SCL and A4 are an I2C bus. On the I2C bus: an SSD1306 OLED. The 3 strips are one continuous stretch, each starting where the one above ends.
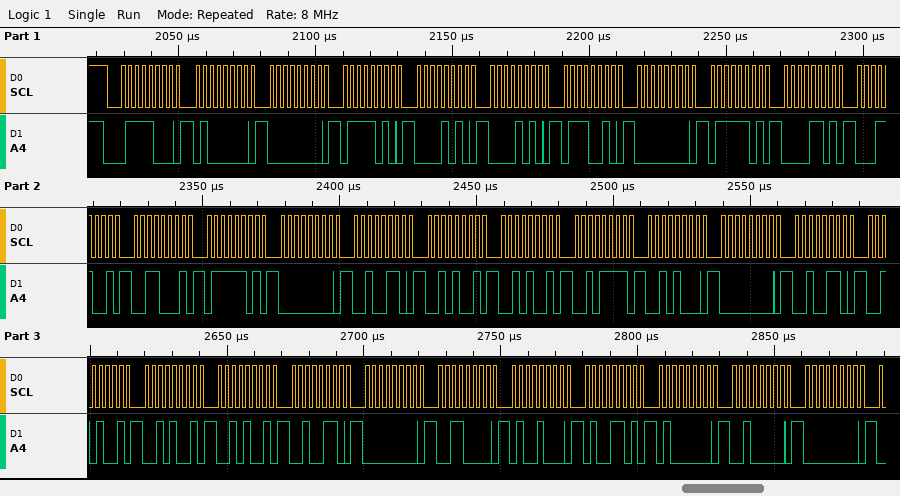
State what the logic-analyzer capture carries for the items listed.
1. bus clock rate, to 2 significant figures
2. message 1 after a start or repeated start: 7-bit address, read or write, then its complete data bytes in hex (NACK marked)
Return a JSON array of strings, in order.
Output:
["400 kHz", "0x3C write: 40 00 7A 0A 0A 72 00 7D 0D 19 31 7D 00 26 29 29 2F 28 00 26 29 29 29 26 00 30 48 4D 40 20 00"]
